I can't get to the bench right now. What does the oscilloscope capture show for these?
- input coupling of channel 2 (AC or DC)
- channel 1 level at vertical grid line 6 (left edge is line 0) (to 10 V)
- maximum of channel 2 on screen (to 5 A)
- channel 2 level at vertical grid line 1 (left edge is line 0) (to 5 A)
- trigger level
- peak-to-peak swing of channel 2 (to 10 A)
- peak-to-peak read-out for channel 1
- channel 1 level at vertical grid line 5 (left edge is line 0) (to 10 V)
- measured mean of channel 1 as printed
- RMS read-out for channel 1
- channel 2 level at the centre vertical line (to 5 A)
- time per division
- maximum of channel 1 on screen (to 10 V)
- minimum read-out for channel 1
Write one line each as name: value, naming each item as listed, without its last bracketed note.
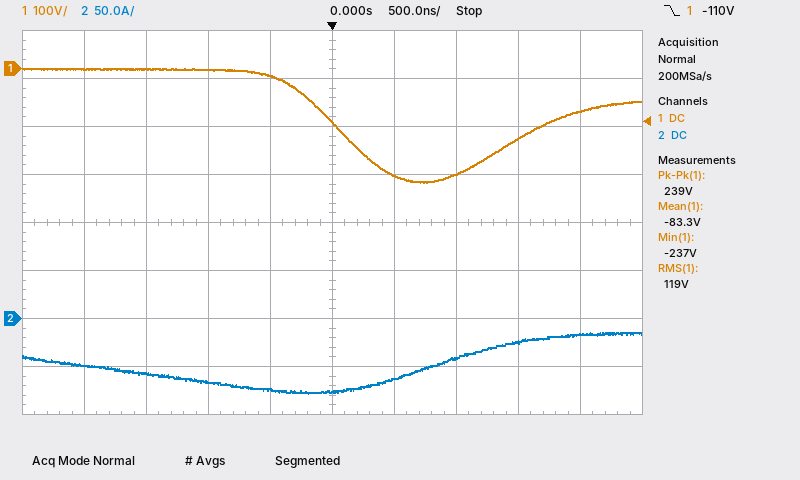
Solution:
input coupling of channel 2: DC
channel 1 level at vertical grid line 6 (left edge is line 0): -220 V
maximum of channel 2 on screen: -15 A
channel 2 level at vertical grid line 1 (left edge is line 0): -50 A
trigger level: -110 V
peak-to-peak swing of channel 2: 60 A
peak-to-peak read-out for channel 1: 239 V
channel 1 level at vertical grid line 5 (left edge is line 0): -110 V
measured mean of channel 1 as printed: -83.3 V
RMS read-out for channel 1: 119 V
channel 2 level at the centre vertical line: -75 A
time per division: 500 ns
maximum of channel 1 on screen: 0 V
minimum read-out for channel 1: -237 V
